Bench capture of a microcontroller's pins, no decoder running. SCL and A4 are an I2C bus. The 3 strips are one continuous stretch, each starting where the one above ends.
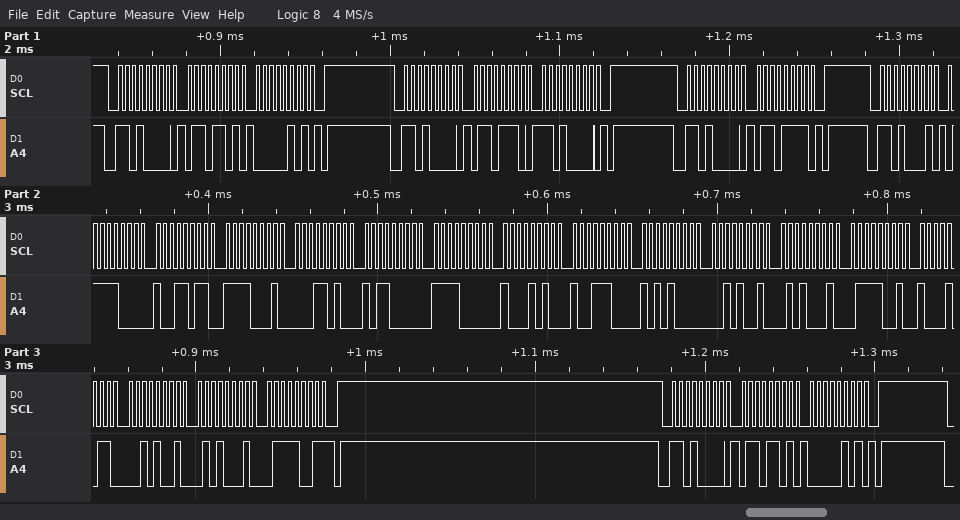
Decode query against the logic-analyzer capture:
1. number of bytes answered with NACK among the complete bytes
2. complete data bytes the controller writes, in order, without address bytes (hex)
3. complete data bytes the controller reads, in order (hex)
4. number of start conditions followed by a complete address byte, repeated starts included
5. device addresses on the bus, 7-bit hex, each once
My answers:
1
6D 05 6E D0 6F 6D 05
78 9B F1 1A B0 F0 8A 9C A8 29 51 79 8B 29 51 79
5
0x68
